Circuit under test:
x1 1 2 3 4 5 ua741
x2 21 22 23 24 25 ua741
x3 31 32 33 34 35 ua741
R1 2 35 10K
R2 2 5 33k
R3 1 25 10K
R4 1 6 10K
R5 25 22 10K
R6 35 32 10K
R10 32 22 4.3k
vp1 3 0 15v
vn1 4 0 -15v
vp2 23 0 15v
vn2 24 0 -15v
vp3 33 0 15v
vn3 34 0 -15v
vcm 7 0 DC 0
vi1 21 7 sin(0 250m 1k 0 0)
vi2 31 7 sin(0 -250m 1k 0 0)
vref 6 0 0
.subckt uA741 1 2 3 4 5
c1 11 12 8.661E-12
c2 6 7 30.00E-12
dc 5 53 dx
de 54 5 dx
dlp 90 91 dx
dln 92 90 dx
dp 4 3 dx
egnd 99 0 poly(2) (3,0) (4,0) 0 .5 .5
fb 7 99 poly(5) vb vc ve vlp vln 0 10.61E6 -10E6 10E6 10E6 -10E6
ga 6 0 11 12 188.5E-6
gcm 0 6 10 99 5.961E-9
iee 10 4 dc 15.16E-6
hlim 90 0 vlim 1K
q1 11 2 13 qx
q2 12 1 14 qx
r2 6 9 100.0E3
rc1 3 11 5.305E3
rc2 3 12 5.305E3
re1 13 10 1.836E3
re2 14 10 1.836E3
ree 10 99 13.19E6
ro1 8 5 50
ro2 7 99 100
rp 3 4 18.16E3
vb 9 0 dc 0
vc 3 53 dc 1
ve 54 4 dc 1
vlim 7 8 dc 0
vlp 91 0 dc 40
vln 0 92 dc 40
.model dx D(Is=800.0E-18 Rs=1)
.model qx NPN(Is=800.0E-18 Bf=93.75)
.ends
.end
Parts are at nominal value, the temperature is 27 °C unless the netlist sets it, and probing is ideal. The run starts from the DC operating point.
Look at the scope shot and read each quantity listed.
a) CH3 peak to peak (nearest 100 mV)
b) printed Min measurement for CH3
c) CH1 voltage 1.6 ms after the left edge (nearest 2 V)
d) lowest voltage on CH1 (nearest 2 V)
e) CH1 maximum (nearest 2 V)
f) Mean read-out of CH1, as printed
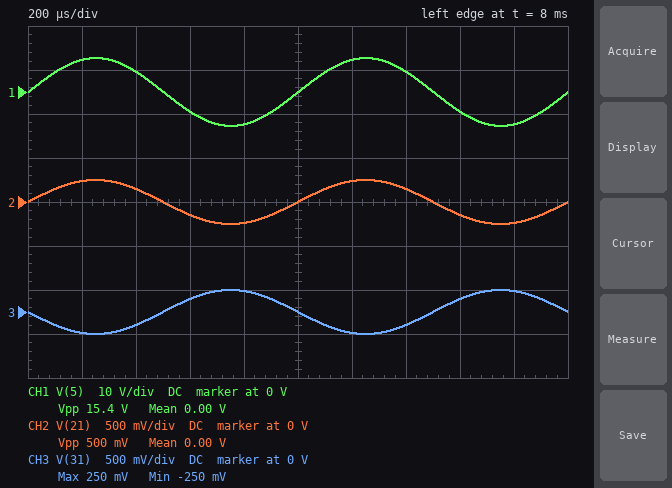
500 mV
-250 mV
-4 V
-8 V
8 V
0.00 V
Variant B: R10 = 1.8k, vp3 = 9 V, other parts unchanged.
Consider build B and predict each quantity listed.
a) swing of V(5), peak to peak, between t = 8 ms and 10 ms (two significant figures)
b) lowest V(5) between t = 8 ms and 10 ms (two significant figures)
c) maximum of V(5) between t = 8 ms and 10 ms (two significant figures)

29 V
-15 V
15 V
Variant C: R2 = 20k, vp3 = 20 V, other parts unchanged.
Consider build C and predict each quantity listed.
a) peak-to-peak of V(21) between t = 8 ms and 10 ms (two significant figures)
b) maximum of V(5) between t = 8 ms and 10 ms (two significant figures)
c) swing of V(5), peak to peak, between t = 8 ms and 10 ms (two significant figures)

500 mV
4.9 V
9.9 V
